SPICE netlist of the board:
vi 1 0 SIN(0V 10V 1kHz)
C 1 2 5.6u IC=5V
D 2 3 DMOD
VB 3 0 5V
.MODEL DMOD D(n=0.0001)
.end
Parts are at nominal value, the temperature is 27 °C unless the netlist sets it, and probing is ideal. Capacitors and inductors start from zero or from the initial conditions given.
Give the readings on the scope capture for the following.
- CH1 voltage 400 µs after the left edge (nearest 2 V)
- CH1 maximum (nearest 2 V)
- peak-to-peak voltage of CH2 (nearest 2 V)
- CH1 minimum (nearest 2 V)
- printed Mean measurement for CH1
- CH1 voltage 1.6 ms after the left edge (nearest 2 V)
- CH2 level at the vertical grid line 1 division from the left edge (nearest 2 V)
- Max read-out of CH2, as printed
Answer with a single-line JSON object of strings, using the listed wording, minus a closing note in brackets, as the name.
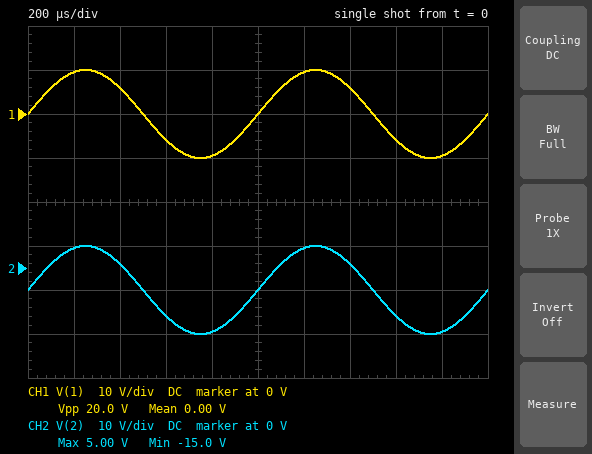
{"CH1 voltage 400 µs after the left edge": "6 V", "CH1 maximum": "10 V", "peak-to-peak voltage of CH2": "20 V", "CH1 minimum": "-10 V", "printed Mean measurement for CH1": "0.00 V", "CH1 voltage 1.6 ms after the left edge": "-6 V", "CH2 level at the vertical grid line 1 division from the left edge": "4 V", "Max read-out of CH2, as printed": "5.00 V"}
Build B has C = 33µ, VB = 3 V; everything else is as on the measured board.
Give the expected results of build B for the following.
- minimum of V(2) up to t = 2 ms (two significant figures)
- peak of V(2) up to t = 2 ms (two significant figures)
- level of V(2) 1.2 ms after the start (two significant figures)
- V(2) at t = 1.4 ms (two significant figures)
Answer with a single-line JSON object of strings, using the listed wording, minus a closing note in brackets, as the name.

{"minimum of V(2) up to t = 2 ms": "-17 V", "peak of V(2) up to t = 2 ms": "3.0 V", "level of V(2) 1.2 ms after the start": "2.5 V", "V(2) at t = 1.4 ms": "-1.1 V"}
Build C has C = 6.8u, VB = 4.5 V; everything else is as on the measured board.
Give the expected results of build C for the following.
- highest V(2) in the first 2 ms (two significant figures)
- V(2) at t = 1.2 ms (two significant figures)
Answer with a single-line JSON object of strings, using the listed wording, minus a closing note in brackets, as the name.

{"highest V(2) in the first 2 ms": "4.5 V", "V(2) at t = 1.2 ms": "4.0 V"}
